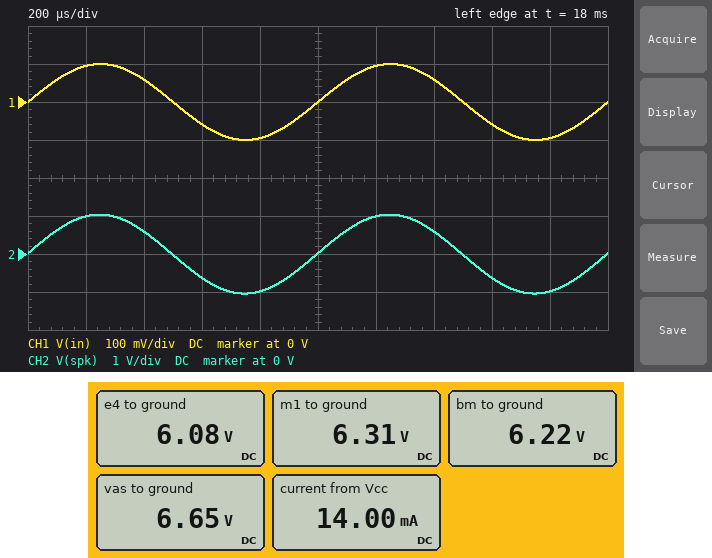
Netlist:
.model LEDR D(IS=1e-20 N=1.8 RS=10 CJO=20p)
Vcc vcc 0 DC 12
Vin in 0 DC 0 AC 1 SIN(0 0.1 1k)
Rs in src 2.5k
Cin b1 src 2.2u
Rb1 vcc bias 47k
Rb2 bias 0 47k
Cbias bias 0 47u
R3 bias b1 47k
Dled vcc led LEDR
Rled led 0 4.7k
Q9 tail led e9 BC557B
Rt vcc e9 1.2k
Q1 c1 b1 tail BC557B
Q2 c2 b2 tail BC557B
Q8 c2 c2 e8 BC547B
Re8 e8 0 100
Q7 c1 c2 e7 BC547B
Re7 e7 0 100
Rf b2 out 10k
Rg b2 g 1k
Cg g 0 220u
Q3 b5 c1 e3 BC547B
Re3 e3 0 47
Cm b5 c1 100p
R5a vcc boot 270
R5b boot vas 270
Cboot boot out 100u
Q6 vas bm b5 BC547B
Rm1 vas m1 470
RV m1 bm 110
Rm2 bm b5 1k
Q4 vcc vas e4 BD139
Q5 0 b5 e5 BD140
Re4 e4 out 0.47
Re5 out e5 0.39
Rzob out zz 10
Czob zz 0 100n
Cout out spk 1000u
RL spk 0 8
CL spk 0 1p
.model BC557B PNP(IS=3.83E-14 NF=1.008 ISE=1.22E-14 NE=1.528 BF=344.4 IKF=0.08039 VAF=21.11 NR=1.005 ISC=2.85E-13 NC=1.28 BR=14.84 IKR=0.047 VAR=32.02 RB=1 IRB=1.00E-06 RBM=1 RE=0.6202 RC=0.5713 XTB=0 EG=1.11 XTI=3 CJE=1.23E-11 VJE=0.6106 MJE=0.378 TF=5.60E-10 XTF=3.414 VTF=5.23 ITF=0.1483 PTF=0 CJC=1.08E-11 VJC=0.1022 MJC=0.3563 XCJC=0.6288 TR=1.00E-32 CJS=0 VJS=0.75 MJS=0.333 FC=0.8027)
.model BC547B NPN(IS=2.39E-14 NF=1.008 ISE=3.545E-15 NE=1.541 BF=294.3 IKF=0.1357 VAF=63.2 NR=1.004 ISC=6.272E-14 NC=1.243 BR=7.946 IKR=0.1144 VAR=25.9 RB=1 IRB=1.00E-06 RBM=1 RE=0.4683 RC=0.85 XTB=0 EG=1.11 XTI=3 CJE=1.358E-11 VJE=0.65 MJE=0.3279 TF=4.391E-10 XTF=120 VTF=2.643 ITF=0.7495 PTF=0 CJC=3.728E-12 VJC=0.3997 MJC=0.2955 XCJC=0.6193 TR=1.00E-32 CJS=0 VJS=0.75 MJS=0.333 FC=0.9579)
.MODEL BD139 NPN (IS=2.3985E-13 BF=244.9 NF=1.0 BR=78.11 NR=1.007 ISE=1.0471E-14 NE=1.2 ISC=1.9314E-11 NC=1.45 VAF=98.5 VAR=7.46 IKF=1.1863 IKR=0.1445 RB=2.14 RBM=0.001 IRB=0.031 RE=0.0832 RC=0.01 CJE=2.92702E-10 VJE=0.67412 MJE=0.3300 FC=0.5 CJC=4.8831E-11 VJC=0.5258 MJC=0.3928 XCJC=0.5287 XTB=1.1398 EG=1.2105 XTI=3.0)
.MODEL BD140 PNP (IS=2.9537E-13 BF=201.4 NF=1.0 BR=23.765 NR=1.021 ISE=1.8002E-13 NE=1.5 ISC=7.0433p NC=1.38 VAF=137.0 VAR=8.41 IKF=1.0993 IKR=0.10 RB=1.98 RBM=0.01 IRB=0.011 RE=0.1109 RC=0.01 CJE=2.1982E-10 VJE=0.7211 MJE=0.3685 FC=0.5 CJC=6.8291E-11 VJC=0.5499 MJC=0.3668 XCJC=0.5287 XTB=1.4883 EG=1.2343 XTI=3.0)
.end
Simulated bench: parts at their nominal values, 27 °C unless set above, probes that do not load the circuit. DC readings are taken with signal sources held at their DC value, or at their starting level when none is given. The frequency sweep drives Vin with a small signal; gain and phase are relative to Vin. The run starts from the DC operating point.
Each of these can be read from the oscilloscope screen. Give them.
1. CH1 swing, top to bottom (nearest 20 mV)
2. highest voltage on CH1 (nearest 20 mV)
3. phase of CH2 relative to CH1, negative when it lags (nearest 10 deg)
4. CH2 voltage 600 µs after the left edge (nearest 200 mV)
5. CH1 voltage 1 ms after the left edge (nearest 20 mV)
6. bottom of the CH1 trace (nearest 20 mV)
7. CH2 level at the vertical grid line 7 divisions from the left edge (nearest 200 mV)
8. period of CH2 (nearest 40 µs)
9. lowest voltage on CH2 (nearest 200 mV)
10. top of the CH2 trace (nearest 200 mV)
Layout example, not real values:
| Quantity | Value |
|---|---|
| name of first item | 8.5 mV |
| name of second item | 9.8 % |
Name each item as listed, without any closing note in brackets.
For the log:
| Quantity | Value |
|---|---|
| CH1 swing, top to bottom | 200 mV |
| highest voltage on CH1 | 100 mV |
| phase of CH2 relative to CH1, negative when it lags | 0 deg |
| CH2 voltage 600 µs after the left edge | -600 mV |
| CH1 voltage 1 ms after the left edge | 0 V |
| bottom of the CH1 trace | -100 mV |
| CH2 level at the vertical grid line 7 divisions from the left edge | 600 mV |
| period of CH2 | 1.00 ms |
| lowest voltage on CH2 | -1.0 V |
| top of the CH2 trace | 1.0 V |
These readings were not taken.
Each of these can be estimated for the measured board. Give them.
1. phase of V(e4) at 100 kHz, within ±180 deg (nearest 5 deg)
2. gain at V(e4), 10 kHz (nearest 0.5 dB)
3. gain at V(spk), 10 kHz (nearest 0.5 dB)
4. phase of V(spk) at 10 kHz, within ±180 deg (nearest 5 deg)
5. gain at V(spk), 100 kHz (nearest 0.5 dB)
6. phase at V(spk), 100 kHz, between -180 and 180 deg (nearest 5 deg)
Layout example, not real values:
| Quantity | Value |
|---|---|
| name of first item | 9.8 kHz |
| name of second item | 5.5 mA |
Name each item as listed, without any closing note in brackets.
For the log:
| Quantity | Value |
|---|---|
| phase of V(e4) at 100 kHz, within ±180 deg | -10 deg |
| gain at V(e4), 10 kHz | 20.5 dB |
| gain at V(spk), 10 kHz | 20.0 dB |
| phase of V(spk) at 10 kHz, within ±180 deg | 0 deg |
| gain at V(spk), 100 kHz | 20.5 dB |
| phase at V(spk), 100 kHz, between -180 and 180 deg | -10 deg |
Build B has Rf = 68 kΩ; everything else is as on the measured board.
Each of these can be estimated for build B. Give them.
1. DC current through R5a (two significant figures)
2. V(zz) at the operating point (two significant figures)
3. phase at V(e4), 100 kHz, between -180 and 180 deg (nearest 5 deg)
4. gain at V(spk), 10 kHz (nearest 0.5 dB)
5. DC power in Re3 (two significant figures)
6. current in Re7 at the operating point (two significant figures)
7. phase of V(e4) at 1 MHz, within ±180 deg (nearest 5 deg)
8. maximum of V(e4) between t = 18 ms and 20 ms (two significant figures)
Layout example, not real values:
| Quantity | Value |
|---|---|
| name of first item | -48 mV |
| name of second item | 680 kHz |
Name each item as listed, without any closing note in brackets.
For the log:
| Quantity | Value |
|---|---|
| DC current through R5a | 10 mA |
| V(zz) at the operating point | 6.0 V |
| phase at V(e4), 100 kHz, between -180 and 180 deg | -55 deg |
| gain at V(spk), 10 kHz | 35.0 dB |
| DC power in Re3 | 4.8 mW |
| current in Re7 at the operating point | 500 µA |
| phase of V(e4) at 1 MHz, within ±180 deg | -130 deg |
| maximum of V(e4) between t = 18 ms and 20 ms | 12 V |
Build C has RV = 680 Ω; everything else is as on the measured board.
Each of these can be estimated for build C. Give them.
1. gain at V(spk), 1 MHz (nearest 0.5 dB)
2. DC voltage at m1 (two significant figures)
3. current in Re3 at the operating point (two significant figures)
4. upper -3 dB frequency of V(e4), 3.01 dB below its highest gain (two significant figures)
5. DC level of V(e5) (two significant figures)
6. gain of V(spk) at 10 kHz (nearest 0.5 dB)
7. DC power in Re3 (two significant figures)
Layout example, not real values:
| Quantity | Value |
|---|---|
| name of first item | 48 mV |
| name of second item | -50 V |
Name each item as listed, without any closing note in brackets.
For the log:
| Quantity | Value |
|---|---|
| gain at V(spk), 1 MHz | 21.5 dB |
| DC voltage at m1 | 6.5 V |
| current in Re3 at the operating point | 9.6 mA |
| upper -3 dB frequency of V(e4), 3.01 dB below its highest gain | 2.4 MHz |
| DC level of V(e5) | 6.0 V |
| gain of V(spk) at 10 kHz | 20.5 dB |
| DC power in Re3 | 4.4 mW |
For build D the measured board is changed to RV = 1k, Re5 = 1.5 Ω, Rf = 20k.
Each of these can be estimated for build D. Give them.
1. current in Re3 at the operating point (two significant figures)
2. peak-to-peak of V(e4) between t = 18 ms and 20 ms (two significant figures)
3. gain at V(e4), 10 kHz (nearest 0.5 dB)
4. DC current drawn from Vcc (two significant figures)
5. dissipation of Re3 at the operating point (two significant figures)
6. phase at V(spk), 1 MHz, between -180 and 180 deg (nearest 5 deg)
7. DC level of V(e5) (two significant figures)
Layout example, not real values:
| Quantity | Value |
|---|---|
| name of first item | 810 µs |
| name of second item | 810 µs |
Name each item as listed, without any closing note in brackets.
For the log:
| Quantity | Value |
|---|---|
| current in Re3 at the operating point | 9.6 mA |
| peak-to-peak of V(e4) between t = 18 ms and 20 ms | 4.1 V |
| gain at V(e4), 10 kHz | 26.5 dB |
| DC current drawn from Vcc | 170 mA |
| dissipation of Re3 at the operating point | 4.4 mW |
| phase at V(spk), 1 MHz, between -180 and 180 deg | -65 deg |
| DC level of V(e5) | 5.8 V |
